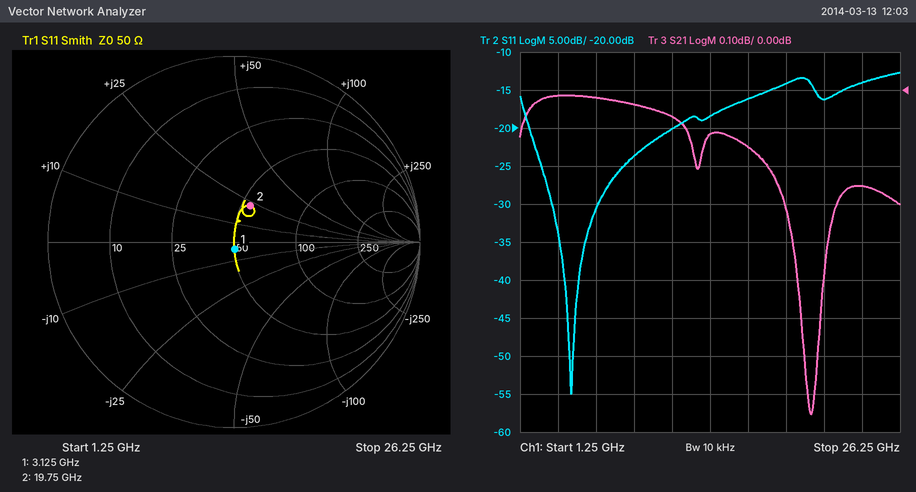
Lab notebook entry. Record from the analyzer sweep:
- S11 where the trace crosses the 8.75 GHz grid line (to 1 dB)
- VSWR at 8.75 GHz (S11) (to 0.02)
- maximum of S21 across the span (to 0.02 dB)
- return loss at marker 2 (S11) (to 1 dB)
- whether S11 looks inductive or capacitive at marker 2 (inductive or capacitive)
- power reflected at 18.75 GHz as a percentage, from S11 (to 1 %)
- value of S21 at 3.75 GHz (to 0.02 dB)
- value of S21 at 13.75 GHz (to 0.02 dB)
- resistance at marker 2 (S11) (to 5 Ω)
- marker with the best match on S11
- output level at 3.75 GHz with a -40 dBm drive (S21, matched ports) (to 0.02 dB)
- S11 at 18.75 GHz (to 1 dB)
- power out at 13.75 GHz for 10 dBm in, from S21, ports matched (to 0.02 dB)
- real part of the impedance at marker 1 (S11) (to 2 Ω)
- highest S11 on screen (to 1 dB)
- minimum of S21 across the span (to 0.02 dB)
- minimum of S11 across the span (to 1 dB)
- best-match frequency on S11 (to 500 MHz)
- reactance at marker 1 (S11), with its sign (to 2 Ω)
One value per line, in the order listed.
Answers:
-24 dB
1.14
-0.02 dB
13 dB
inductive
4 %
-0.02 dB
-0.12 dB
55 Ω
marker 1
-40.02 dBm
-14 dB
9.88 dBm
50 Ω
-13 dB
-0.86 dB
-55 dB
4.5 GHz
-4 Ω
